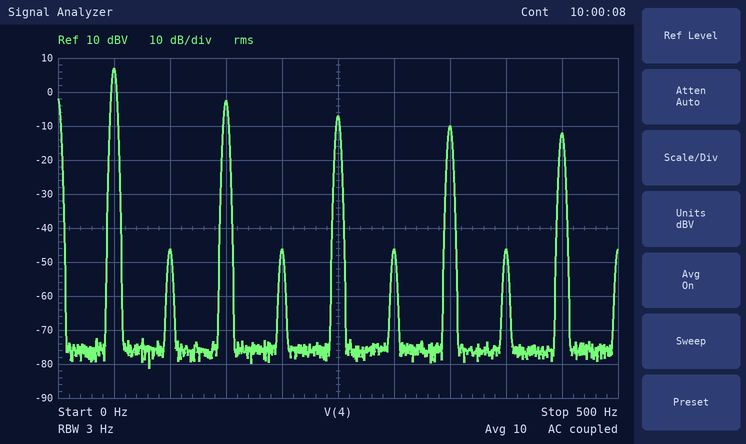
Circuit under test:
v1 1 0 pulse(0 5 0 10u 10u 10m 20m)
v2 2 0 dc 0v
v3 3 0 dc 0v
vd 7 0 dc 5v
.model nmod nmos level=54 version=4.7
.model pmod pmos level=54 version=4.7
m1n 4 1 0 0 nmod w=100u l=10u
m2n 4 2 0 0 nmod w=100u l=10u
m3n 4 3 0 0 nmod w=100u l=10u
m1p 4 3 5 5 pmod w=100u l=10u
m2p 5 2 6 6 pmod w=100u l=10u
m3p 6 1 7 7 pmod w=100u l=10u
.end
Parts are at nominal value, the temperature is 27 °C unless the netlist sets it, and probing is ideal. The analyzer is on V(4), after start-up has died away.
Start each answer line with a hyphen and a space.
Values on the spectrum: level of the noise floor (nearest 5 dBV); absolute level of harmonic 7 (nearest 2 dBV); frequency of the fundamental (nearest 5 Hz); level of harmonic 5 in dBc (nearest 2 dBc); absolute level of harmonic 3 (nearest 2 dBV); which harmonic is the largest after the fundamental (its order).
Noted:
- -75 dBV
- -10 dBV
- 50 Hz
- -14 dBc
- -2 dBV
- 3
